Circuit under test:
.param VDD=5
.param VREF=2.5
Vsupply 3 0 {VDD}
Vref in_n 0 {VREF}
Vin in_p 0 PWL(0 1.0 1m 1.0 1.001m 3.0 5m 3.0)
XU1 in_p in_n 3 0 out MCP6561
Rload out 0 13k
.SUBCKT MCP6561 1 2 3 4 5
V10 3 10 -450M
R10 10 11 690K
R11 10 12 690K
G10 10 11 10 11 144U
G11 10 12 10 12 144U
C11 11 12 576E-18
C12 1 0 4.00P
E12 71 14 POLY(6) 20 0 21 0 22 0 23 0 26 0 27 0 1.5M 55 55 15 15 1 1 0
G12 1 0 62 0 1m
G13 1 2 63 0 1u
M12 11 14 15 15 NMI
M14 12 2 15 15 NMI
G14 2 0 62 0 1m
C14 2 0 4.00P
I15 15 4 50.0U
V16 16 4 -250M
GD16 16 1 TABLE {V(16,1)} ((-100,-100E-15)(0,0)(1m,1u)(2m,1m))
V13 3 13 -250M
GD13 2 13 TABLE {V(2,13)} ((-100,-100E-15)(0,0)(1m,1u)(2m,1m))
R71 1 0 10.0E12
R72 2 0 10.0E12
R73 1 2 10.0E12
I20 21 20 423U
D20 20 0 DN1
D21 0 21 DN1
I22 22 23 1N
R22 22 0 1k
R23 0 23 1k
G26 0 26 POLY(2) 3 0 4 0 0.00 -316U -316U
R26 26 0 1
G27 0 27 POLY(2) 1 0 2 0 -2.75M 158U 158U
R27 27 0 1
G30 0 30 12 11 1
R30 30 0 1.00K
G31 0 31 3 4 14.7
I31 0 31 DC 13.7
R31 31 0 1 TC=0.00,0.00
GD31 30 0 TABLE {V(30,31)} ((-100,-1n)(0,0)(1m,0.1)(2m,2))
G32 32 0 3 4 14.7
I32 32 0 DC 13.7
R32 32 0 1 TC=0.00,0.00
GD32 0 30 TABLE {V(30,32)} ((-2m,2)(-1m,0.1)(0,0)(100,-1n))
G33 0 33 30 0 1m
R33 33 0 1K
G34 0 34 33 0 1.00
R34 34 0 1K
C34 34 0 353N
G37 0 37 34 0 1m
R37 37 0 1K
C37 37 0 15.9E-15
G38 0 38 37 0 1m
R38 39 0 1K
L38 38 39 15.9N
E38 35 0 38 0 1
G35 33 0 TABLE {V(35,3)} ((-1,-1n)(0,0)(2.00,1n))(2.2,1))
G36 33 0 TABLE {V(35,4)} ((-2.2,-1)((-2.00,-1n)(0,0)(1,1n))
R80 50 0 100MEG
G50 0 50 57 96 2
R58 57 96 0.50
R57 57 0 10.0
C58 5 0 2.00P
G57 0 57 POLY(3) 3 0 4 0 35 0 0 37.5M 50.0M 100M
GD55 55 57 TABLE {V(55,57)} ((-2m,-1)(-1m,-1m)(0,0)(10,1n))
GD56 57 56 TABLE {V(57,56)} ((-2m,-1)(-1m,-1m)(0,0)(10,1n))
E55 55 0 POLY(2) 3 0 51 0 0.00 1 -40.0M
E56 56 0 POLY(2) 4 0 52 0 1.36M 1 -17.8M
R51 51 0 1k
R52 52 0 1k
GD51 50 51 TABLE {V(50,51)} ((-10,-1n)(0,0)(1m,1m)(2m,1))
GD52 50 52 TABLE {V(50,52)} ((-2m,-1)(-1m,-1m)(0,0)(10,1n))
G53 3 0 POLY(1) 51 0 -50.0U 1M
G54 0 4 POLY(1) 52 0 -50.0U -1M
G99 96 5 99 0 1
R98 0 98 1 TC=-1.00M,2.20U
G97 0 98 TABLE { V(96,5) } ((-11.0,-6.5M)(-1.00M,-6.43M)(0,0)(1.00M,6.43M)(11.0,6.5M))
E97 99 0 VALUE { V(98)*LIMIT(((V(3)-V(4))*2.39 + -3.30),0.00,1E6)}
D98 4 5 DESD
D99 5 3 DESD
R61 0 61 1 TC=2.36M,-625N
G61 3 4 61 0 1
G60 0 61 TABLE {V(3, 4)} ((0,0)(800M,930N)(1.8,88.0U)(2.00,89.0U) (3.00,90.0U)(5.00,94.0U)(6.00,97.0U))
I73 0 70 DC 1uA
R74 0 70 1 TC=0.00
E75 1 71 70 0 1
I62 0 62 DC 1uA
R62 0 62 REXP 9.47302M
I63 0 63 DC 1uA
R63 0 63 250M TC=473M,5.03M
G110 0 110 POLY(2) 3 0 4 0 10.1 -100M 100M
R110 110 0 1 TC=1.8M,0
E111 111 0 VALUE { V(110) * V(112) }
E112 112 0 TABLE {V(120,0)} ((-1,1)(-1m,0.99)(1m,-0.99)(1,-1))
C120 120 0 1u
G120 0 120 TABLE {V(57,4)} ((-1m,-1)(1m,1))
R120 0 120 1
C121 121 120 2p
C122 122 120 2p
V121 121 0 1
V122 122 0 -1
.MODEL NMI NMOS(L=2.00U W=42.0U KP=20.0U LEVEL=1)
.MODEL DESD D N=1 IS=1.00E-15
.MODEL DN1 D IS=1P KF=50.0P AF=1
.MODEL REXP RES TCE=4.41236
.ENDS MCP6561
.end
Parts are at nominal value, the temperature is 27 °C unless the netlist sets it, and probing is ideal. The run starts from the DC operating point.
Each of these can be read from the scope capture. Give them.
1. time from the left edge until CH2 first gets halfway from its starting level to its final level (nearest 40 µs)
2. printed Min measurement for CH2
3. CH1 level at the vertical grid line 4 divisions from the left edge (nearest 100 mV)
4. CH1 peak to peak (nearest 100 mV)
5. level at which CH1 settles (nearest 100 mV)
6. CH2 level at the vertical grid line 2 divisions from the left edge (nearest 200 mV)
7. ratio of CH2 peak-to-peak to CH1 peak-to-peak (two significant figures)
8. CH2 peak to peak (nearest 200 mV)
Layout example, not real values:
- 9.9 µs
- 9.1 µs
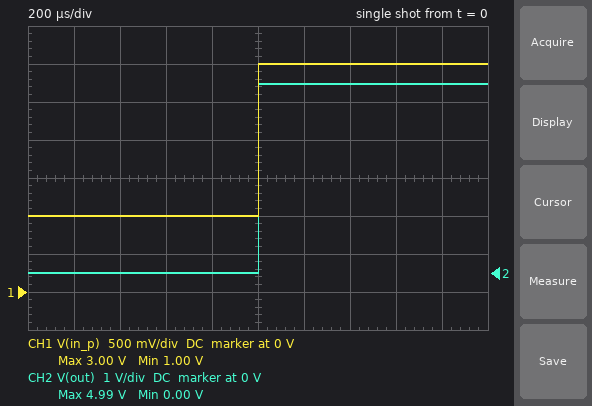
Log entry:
- 1.00 ms
- 0.00 V
- 1.0 V
- 2.0 V
- 3.0 V
- 0 V
- 2.5
- 5.0 V
